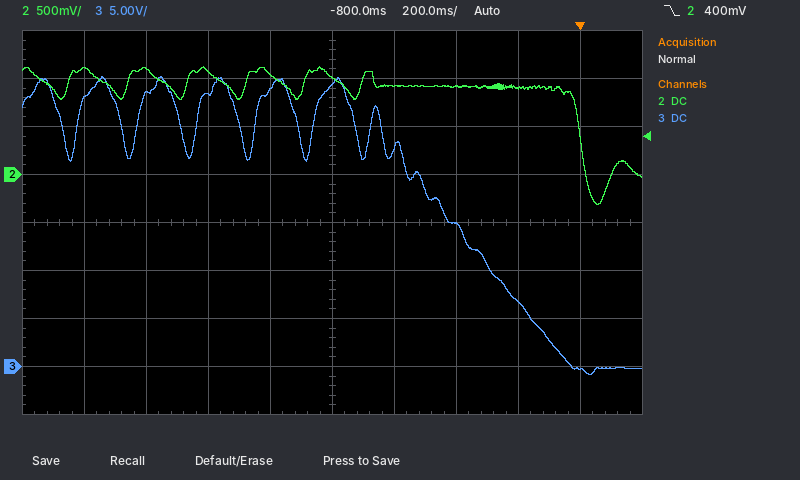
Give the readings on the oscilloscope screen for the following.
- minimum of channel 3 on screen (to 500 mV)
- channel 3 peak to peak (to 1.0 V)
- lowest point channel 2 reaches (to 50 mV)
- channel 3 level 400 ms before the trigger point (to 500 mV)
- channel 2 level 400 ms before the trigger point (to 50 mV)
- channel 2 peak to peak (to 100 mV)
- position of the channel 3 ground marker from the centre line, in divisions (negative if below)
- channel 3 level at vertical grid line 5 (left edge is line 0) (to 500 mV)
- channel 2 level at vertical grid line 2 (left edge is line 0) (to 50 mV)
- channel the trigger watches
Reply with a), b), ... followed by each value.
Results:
a) -1.0 V
b) 31.0 V
c) -300 mV
d) 15.0 V
e) 900 mV
f) 1.40 V
g) -3.0 div
h) 29.5 V
i) 1.10 V
j) channel 2
